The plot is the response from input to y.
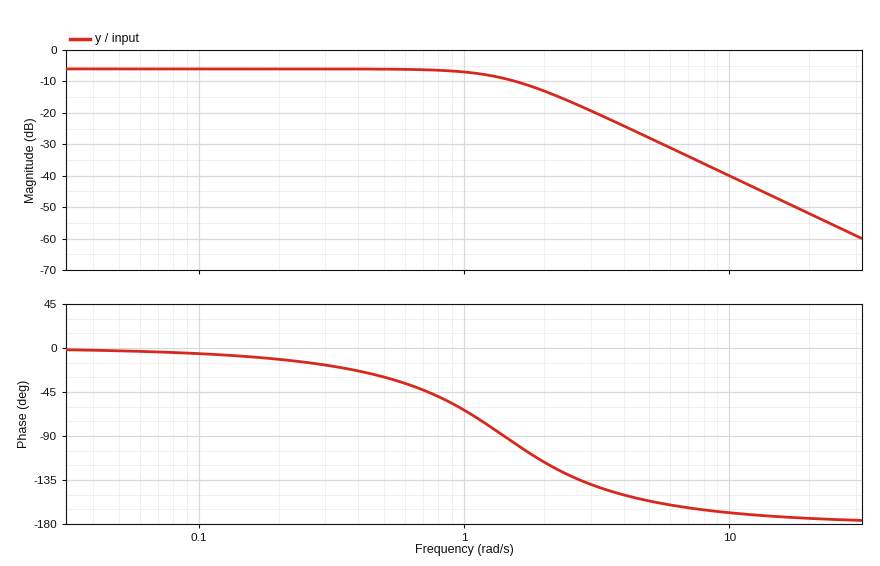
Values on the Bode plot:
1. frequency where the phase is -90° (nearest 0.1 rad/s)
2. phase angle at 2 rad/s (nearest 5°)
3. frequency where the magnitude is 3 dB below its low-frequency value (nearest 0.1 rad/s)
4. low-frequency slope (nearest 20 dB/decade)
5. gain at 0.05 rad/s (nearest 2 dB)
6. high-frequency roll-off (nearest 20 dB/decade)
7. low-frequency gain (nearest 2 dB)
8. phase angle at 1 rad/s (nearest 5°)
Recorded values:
1.4 rad/s
-115°
1.4 rad/s
0 dB/decade
-6 dB
-40 dB/decade
-6 dB
-65°
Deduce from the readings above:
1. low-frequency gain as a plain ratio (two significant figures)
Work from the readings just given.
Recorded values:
0.50
